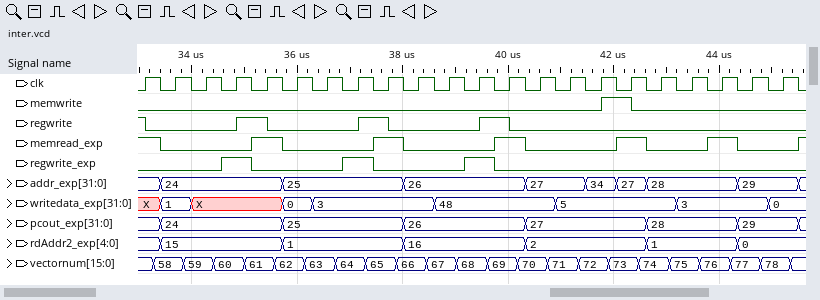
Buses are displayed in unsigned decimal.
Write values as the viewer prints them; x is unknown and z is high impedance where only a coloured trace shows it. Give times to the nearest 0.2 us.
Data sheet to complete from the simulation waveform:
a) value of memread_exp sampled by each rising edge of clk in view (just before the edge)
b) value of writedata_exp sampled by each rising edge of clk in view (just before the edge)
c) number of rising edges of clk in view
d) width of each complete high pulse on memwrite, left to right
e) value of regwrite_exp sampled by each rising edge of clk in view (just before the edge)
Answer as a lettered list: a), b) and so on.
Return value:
a) 1 0 0 0 1 0 0 0 1 0 0 0 1 0 0 0 1 0 0 1 0 0
b) X, 1, X, X, X, 0, 3, 3, 3, 3, 48, 48, 48, 48, 5, 5, 5, 5, 3, 3, 3, 0
c) 22
d) 0.6 us
e) 0 0 0 1 0 0 0 1 0 0 0 1 0 0 0 0 0 0 0 0 0 0
